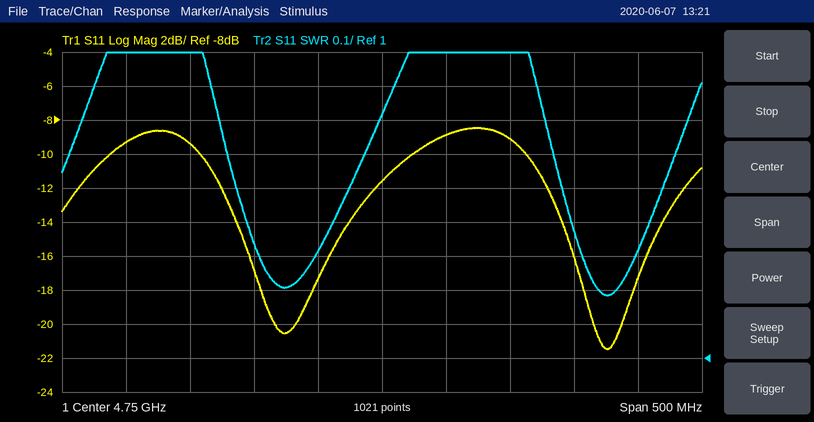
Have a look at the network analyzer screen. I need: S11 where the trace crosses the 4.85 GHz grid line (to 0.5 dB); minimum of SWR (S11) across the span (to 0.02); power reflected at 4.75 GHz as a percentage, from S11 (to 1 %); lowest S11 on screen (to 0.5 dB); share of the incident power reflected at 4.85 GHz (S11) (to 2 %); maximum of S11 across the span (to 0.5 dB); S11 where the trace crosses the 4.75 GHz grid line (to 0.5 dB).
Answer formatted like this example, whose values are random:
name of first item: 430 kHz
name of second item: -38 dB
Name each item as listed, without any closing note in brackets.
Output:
S11 where the trace crosses the 4.85 GHz grid line: -9.0 dB
minimum of SWR (S11) across the span: 1.18
power reflected at 4.75 GHz as a percentage, from S11: 7 %
lowest S11 on screen: -21.5 dB
share of the incident power reflected at 4.85 GHz (S11): 12 %
maximum of S11 across the span: -8.5 dB
S11 where the trace crosses the 4.75 GHz grid line: -11.5 dB
